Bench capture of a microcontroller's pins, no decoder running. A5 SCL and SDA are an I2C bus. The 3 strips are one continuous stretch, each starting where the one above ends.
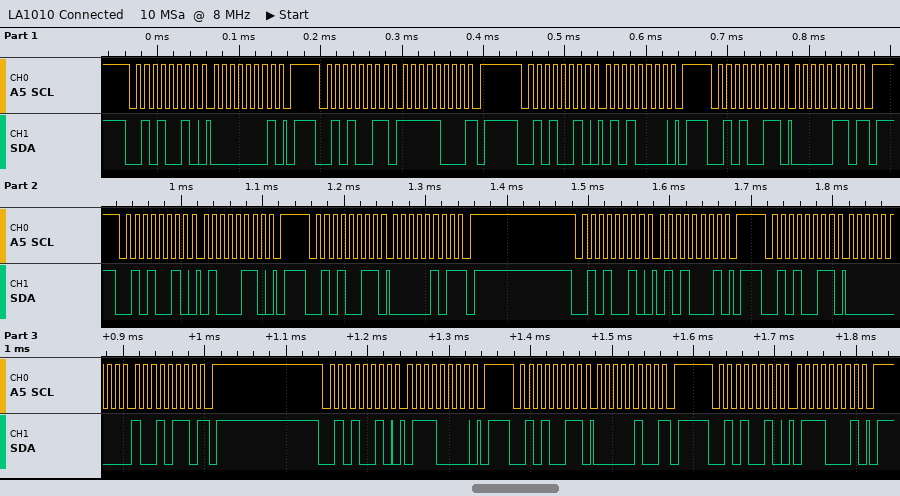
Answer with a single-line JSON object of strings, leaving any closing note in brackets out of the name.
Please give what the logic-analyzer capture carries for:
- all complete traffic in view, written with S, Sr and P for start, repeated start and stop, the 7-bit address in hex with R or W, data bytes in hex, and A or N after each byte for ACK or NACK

{"all complete traffic in view, written with S, Sr and P for start, repeated start and stop, the 7-bit address in hex with R or W, data bytes in hex, and A or N after each byte for ACK or NACK": "S 29W A 01 A P S 29R A F8 N P S 29W A 50 A P S 29R A 06 N P S 29W A 46 A P S 29R A 05 N P S 29W A 51 A P S 29R A 00 A 96 N P S 29W A 70 A P S 29R A 04 N P S 29W A 71 A P"}
